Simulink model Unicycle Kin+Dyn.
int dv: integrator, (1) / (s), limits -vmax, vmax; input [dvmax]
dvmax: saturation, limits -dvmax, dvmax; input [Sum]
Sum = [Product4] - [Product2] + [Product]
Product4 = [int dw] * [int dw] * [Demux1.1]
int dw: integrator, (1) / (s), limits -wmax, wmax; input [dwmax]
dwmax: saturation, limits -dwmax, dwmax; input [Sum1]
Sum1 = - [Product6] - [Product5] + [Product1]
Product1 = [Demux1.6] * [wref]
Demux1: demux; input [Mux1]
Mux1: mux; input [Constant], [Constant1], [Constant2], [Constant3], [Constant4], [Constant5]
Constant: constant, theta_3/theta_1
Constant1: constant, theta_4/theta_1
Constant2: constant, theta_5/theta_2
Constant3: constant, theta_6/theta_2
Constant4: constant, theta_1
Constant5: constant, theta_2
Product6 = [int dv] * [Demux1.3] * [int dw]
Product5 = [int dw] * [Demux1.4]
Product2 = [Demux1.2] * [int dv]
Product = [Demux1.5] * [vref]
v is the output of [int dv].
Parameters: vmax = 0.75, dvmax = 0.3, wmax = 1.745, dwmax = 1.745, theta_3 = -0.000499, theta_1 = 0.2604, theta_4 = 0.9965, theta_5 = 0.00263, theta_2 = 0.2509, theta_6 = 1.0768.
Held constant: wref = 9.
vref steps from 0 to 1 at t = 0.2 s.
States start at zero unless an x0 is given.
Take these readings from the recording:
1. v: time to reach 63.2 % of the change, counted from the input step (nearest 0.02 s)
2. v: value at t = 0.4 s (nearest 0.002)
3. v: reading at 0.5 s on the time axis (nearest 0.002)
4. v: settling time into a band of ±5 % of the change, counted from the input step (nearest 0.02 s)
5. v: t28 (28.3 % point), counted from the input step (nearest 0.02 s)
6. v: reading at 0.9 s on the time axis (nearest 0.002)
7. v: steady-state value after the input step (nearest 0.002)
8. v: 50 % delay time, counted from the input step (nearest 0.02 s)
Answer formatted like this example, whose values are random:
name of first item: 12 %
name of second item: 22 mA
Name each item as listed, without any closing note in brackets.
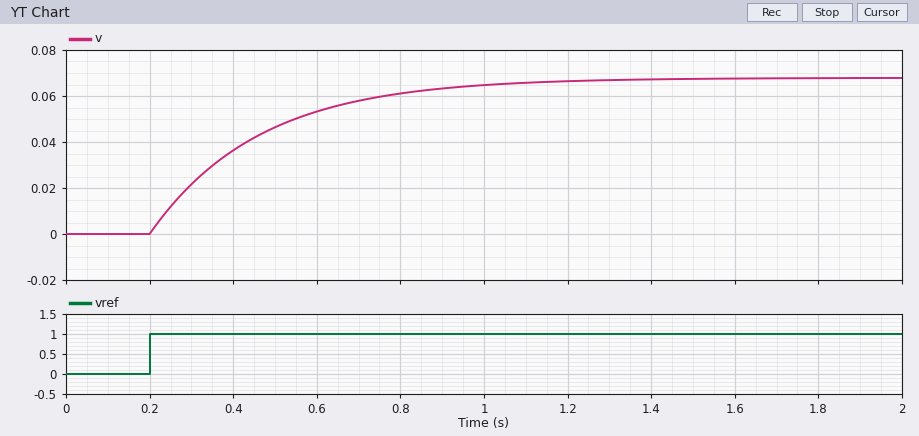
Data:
v: time to reach 63.2 % of the change, counted from the input step: 0.26 s
v: value at t = 0.4 s: 0.036
v: reading at 0.5 s on the time axis: 0.046
v: settling time into a band of ±5 % of the change, counted from the input step: 0.78 s
v: t28 (28.3 % point), counted from the input step: 0.08 s
v: reading at 0.9 s on the time axis: 0.064
v: steady-state value after the input step: 0.068
v: 50 % delay time, counted from the input step: 0.18 s
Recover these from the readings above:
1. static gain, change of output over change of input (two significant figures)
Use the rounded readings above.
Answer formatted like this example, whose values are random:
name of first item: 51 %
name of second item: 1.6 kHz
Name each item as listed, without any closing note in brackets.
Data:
static gain, change of output over change of input: 0.068
